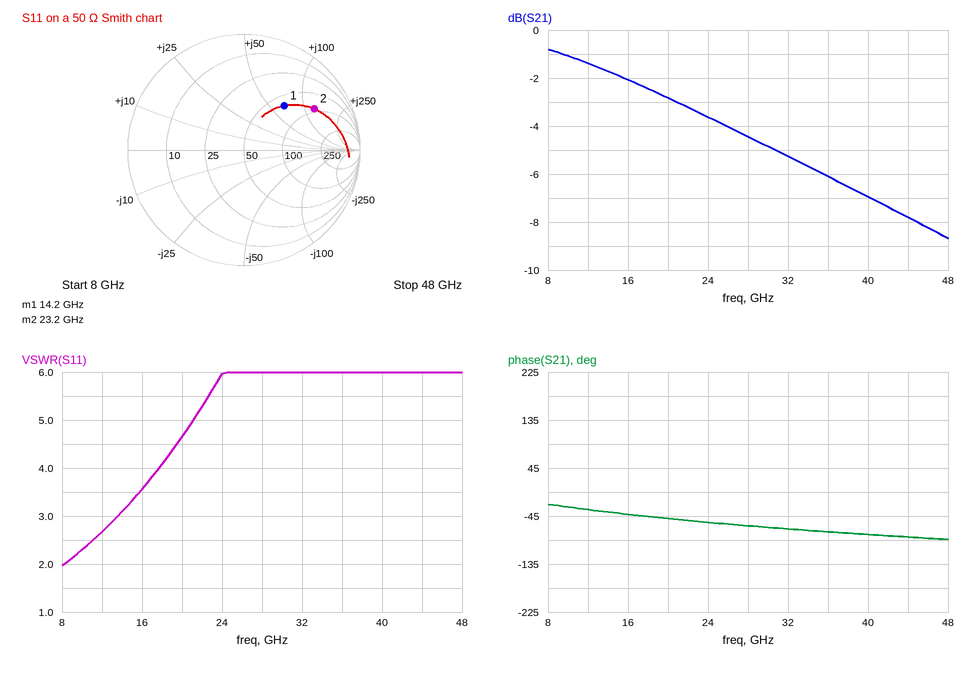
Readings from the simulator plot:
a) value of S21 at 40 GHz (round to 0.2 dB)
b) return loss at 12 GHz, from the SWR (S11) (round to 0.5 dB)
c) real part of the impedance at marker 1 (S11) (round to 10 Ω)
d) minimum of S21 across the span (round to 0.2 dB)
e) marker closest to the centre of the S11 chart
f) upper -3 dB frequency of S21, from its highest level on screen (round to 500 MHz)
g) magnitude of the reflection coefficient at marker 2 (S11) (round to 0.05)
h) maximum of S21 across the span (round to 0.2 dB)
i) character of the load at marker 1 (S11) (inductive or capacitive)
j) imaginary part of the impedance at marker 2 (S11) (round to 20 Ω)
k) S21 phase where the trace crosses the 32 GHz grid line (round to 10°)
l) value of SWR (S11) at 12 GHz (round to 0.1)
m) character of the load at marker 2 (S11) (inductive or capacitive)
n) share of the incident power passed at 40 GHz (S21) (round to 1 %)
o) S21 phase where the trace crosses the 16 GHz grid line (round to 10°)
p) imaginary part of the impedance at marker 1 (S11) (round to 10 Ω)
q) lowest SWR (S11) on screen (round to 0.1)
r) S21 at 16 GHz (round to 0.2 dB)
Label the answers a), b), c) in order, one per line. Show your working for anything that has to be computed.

a) -7.0 dB
b) −20 log10((2.7 − 1)/(2.7 + 1)) ≈ 6.76 dB, so 7.0 dB to the nearest 0.5 dB
c) 60 Ω
d) -8.6 dB
e) marker 1
f) 25.0 GHz
g) 0.70
h) -0.8 dB
i) inductive
j) +120 Ω
k) -70°
l) 2.7
m) inductive
n) 10^(-7/10) ≈ 20 %
o) -40°
p) +70 Ω
q) 2.0
r) -2.0 dB
